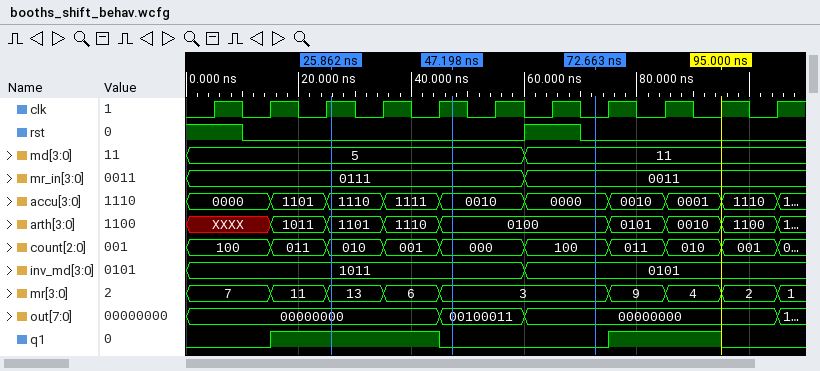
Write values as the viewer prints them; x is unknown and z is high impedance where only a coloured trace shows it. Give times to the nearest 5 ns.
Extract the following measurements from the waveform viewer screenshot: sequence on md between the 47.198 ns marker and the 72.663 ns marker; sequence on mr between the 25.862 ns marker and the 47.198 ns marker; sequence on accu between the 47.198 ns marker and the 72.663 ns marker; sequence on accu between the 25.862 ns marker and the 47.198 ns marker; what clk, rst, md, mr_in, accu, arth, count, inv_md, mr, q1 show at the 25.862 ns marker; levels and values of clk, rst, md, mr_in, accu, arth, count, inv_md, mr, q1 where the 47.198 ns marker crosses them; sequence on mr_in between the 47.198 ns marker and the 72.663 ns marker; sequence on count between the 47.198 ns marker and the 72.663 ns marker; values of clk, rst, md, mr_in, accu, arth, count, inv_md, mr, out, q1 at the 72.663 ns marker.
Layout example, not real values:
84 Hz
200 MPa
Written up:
5, 11
13, 6, 3
0010, 0000
1110, 1111, 0010
clk=1, rst=0, md=5, mr_in=0111, accu=1110, arth=1101, count=010, inv_md=1011, mr=13, q1=1
clk=1, rst=0, md=5, mr_in=0111, accu=0010, arth=0100, count=000, inv_md=1011, mr=3, q1=0
0111, 0011
000, 100
clk=0, rst=0, md=11, mr_in=0011, accu=0000, arth=0100, count=100, inv_md=0101, mr=3, out=00000000, q1=0
